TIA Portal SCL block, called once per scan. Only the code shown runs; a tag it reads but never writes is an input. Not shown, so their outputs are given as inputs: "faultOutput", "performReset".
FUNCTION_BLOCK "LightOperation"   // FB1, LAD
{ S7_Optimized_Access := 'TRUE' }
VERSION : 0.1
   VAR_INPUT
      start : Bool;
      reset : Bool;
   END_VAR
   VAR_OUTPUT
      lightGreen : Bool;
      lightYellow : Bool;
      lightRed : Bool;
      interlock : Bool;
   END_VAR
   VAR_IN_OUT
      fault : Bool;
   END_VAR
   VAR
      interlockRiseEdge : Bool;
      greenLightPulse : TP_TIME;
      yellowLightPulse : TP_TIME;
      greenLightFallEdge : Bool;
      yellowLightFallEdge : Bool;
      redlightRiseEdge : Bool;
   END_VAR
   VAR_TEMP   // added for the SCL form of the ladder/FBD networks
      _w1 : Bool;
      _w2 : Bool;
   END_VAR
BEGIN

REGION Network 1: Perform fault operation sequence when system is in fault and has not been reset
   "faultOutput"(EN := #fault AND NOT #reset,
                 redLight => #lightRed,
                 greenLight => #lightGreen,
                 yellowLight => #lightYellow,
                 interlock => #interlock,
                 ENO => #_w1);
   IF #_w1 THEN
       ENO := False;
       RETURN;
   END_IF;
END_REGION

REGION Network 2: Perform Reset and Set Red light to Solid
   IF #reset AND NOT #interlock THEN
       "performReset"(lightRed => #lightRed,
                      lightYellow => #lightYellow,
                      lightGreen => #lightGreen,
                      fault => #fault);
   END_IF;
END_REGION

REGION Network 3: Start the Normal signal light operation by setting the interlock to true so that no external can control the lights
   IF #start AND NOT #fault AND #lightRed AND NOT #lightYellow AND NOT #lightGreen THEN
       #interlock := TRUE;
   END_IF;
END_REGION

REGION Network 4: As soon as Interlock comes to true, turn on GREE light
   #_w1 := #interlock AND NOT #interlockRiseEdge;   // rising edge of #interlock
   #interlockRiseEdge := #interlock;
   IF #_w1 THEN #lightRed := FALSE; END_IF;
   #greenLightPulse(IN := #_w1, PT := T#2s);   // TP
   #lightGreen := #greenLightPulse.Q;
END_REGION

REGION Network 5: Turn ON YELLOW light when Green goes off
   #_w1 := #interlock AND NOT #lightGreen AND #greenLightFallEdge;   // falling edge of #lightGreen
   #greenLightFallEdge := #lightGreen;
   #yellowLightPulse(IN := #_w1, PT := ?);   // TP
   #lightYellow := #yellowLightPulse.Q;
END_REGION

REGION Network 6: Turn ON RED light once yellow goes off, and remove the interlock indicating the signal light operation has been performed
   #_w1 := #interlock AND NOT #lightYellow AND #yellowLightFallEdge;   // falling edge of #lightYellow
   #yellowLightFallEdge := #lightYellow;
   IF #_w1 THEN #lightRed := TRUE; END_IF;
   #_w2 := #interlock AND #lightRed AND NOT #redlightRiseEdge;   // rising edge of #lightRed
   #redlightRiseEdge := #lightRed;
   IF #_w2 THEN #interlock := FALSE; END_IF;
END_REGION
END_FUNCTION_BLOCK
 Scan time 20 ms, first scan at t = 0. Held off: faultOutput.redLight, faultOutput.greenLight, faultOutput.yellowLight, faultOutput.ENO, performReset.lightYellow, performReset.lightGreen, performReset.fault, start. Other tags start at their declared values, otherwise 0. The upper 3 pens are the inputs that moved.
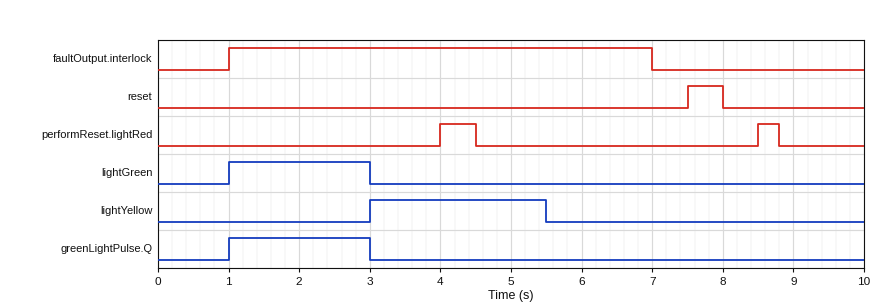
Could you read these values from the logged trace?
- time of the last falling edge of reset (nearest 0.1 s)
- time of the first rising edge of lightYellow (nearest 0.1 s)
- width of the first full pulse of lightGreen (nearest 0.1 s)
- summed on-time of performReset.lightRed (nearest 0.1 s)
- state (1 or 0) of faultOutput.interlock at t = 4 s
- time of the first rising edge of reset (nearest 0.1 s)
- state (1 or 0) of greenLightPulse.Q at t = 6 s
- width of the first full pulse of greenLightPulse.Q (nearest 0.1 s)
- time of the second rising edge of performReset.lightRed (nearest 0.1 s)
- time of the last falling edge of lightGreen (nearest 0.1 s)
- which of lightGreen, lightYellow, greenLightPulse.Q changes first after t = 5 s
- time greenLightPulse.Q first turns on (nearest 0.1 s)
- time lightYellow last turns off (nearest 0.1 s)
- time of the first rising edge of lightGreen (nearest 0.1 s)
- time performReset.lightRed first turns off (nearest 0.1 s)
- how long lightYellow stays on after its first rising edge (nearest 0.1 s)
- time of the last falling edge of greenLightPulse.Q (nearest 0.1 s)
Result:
8.0 s
3.0 s
2.0 s
0.8 s
1
7.5 s
0
2.0 s
8.5 s
3.0 s
lightYellow
1.0 s
5.5 s
1.0 s
4.5 s
2.5 s
3.0 s
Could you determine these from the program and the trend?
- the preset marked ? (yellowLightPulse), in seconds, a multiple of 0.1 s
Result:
2.5 s
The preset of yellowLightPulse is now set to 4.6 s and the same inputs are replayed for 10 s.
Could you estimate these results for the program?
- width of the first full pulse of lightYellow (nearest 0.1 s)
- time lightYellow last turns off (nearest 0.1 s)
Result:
4.6 s
7.6 s
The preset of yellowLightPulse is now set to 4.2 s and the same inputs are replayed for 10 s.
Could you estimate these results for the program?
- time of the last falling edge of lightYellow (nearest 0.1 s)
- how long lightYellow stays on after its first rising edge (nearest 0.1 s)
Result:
7.2 s
4.2 s
